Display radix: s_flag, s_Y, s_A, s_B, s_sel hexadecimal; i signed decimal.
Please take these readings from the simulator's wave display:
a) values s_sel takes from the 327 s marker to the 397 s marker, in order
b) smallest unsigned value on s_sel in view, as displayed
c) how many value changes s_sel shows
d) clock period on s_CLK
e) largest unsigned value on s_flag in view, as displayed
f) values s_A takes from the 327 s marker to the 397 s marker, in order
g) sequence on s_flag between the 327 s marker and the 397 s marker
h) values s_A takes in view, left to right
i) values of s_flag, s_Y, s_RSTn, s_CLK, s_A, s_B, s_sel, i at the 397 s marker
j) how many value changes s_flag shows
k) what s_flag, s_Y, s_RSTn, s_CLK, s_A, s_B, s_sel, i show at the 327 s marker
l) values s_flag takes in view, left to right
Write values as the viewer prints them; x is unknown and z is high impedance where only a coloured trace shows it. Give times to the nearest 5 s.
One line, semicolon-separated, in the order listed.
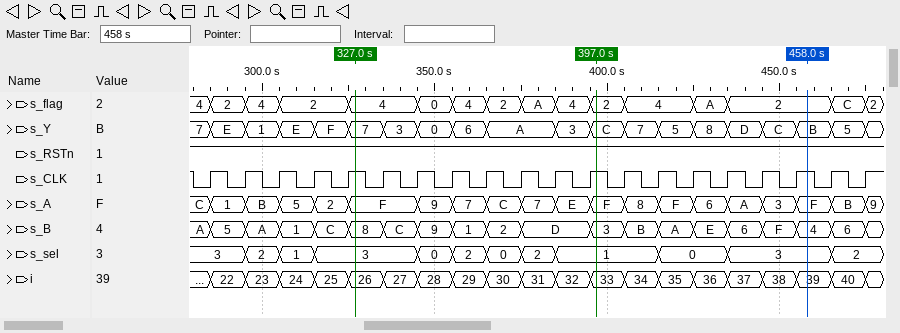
3, 0, 2, 0, 2, 1; 0; 11; 10 s; C; F, 9, 7, C, 7, E, F; 4, 0, 4, 2, A, 4, 2; C, 1, B, 5, 2, F, 9, 7, C, 7, E, F, 8, F, 6, A, 3, F, B, 9; s_flag=2, s_Y=C, s_RSTn=1, s_CLK=1, s_A=F, s_B=3, s_sel=1, i=33; 15; s_flag=4, s_Y=7, s_RSTn=1, s_CLK=1, s_A=F, s_B=8, s_sel=3, i=26; 4, 2, 4, 2, 4, 0, 4, 2, A, 4, 2, 4, A, 2, C, 2
